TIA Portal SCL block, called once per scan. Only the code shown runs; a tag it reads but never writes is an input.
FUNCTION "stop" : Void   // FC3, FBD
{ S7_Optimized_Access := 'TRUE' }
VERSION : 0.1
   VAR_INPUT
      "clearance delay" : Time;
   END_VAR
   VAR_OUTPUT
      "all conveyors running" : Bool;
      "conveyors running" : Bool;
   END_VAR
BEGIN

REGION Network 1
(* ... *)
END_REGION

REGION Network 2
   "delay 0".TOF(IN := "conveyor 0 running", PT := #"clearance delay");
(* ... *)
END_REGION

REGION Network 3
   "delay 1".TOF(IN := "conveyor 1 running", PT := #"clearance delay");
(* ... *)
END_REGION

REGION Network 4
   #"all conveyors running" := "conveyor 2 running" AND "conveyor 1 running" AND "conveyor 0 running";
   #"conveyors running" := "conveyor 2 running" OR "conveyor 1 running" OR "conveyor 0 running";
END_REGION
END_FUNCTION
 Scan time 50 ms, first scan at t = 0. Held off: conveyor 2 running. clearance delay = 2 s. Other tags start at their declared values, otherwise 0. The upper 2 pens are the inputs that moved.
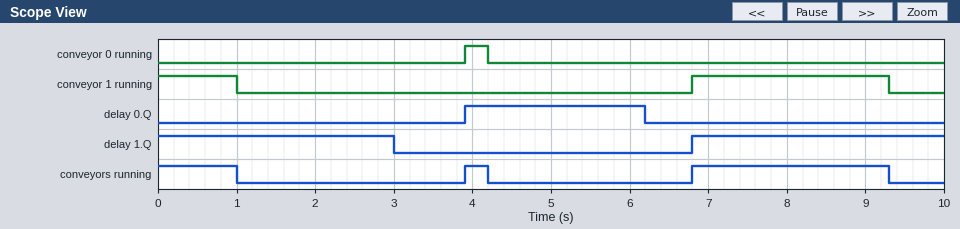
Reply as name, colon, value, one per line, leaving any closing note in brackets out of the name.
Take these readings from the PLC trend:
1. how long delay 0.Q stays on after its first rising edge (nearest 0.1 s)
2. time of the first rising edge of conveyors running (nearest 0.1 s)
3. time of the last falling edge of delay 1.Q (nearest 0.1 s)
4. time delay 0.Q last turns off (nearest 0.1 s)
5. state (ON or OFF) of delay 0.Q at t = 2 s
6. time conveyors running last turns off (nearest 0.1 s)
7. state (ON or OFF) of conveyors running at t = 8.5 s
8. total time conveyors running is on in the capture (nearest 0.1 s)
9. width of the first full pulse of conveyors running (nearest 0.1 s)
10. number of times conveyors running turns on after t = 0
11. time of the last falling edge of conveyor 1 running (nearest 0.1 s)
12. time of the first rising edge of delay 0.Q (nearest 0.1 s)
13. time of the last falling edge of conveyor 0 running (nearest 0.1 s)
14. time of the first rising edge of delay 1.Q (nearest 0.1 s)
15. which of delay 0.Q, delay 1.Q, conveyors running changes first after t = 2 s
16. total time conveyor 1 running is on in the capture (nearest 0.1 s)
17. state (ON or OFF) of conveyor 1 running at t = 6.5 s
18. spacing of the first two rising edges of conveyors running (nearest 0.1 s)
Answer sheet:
how long delay 0.Q stays on after its first rising edge: 2.3 s
time of the first rising edge of conveyors running: 3.9 s
time of the last falling edge of delay 1.Q: 3.0 s
time delay 0.Q last turns off: 6.2 s
state (ON or OFF) of delay 0.Q at t = 2 s: OFF
time conveyors running last turns off: 9.3 s
state (ON or OFF) of conveyors running at t = 8.5 s: ON
total time conveyors running is on in the capture: 3.8 s
width of the first full pulse of conveyors running: 0.3 s
number of times conveyors running turns on after t = 0: 2
time of the last falling edge of conveyor 1 running: 9.3 s
time of the first rising edge of delay 0.Q: 3.9 s
time of the last falling edge of conveyor 0 running: 4.2 s
time of the first rising edge of delay 1.Q: 6.8 s
which of delay 0.Q, delay 1.Q, conveyors running changes first after t = 2 s: delay 1.Q
total time conveyor 1 running is on in the capture: 3.5 s
state (ON or OFF) of conveyor 1 running at t = 6.5 s: OFF
spacing of the first two rising edges of conveyors running: 2.9 s
